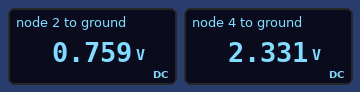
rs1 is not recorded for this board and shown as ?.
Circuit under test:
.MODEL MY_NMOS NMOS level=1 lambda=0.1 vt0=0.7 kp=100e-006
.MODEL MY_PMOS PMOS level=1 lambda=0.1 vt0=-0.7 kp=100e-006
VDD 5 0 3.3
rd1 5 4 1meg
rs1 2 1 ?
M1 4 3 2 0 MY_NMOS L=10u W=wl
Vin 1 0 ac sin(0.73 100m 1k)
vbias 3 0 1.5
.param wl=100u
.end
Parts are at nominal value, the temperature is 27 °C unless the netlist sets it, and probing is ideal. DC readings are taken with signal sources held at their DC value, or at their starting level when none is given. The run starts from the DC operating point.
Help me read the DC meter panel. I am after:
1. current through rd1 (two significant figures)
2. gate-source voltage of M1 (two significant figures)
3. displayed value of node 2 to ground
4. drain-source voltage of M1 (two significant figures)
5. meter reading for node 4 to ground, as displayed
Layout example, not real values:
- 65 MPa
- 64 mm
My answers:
- 970 nA
- 740 mV
- 0.759 V
- 1.6 V
- 2.331 V
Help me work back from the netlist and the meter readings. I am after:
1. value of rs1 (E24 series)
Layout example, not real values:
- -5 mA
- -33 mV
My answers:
- 30 kΩ
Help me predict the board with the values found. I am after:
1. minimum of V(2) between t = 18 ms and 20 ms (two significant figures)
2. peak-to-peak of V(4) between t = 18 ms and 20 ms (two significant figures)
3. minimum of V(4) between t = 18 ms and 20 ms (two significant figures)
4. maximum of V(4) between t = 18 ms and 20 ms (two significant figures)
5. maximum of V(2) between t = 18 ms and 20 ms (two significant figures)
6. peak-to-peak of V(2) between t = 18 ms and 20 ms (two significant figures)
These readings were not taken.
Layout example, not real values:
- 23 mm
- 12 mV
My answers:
- 710 mV
- 2.6 V
- 740 mV
- 3.3 V
- 830 mV
- 120 mV
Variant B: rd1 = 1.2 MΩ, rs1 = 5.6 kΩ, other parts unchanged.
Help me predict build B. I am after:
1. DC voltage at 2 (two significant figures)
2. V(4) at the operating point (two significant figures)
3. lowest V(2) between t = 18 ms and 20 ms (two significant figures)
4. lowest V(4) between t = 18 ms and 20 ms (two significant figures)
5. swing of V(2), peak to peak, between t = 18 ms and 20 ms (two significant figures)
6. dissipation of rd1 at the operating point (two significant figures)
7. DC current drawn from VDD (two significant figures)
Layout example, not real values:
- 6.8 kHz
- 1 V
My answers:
- 740 mV
- 1.1 V
- 640 mV
- 660 mV
- 190 mV
- 4.1 µW
- 1.8 µA
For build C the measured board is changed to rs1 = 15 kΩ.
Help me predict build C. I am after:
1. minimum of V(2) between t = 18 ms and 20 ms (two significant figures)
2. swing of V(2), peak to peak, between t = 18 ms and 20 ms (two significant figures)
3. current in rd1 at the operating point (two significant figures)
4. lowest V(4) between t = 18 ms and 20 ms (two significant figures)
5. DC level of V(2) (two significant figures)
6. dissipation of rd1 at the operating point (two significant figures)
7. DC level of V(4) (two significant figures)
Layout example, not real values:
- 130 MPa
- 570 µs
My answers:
- 670 mV
- 160 mV
- 1.4 µA
- 690 mV
- 750 mV
- 1.9 µW
- 1.9 V
